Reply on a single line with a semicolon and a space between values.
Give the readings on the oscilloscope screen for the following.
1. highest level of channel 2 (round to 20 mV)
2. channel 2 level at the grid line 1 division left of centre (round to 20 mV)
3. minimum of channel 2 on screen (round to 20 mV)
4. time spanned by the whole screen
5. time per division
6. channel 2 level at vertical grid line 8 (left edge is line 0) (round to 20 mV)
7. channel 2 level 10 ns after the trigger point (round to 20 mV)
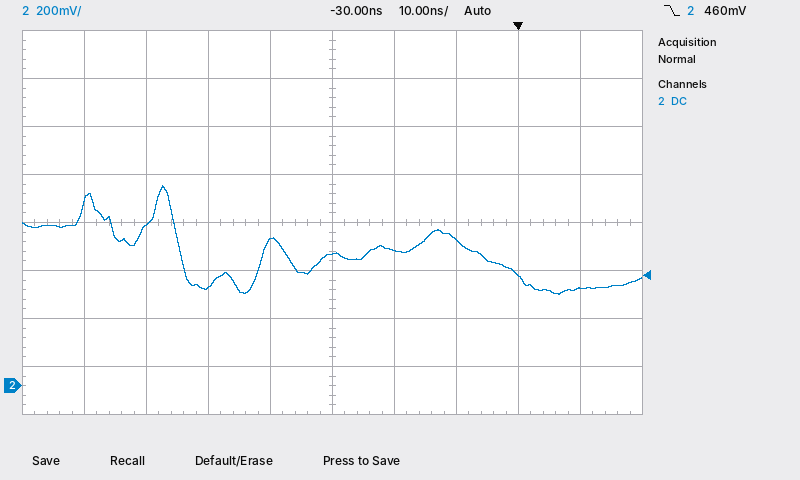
840 mV; 600 mV; 380 mV; 100 ns; 10 ns; 460 mV; 400 mV
